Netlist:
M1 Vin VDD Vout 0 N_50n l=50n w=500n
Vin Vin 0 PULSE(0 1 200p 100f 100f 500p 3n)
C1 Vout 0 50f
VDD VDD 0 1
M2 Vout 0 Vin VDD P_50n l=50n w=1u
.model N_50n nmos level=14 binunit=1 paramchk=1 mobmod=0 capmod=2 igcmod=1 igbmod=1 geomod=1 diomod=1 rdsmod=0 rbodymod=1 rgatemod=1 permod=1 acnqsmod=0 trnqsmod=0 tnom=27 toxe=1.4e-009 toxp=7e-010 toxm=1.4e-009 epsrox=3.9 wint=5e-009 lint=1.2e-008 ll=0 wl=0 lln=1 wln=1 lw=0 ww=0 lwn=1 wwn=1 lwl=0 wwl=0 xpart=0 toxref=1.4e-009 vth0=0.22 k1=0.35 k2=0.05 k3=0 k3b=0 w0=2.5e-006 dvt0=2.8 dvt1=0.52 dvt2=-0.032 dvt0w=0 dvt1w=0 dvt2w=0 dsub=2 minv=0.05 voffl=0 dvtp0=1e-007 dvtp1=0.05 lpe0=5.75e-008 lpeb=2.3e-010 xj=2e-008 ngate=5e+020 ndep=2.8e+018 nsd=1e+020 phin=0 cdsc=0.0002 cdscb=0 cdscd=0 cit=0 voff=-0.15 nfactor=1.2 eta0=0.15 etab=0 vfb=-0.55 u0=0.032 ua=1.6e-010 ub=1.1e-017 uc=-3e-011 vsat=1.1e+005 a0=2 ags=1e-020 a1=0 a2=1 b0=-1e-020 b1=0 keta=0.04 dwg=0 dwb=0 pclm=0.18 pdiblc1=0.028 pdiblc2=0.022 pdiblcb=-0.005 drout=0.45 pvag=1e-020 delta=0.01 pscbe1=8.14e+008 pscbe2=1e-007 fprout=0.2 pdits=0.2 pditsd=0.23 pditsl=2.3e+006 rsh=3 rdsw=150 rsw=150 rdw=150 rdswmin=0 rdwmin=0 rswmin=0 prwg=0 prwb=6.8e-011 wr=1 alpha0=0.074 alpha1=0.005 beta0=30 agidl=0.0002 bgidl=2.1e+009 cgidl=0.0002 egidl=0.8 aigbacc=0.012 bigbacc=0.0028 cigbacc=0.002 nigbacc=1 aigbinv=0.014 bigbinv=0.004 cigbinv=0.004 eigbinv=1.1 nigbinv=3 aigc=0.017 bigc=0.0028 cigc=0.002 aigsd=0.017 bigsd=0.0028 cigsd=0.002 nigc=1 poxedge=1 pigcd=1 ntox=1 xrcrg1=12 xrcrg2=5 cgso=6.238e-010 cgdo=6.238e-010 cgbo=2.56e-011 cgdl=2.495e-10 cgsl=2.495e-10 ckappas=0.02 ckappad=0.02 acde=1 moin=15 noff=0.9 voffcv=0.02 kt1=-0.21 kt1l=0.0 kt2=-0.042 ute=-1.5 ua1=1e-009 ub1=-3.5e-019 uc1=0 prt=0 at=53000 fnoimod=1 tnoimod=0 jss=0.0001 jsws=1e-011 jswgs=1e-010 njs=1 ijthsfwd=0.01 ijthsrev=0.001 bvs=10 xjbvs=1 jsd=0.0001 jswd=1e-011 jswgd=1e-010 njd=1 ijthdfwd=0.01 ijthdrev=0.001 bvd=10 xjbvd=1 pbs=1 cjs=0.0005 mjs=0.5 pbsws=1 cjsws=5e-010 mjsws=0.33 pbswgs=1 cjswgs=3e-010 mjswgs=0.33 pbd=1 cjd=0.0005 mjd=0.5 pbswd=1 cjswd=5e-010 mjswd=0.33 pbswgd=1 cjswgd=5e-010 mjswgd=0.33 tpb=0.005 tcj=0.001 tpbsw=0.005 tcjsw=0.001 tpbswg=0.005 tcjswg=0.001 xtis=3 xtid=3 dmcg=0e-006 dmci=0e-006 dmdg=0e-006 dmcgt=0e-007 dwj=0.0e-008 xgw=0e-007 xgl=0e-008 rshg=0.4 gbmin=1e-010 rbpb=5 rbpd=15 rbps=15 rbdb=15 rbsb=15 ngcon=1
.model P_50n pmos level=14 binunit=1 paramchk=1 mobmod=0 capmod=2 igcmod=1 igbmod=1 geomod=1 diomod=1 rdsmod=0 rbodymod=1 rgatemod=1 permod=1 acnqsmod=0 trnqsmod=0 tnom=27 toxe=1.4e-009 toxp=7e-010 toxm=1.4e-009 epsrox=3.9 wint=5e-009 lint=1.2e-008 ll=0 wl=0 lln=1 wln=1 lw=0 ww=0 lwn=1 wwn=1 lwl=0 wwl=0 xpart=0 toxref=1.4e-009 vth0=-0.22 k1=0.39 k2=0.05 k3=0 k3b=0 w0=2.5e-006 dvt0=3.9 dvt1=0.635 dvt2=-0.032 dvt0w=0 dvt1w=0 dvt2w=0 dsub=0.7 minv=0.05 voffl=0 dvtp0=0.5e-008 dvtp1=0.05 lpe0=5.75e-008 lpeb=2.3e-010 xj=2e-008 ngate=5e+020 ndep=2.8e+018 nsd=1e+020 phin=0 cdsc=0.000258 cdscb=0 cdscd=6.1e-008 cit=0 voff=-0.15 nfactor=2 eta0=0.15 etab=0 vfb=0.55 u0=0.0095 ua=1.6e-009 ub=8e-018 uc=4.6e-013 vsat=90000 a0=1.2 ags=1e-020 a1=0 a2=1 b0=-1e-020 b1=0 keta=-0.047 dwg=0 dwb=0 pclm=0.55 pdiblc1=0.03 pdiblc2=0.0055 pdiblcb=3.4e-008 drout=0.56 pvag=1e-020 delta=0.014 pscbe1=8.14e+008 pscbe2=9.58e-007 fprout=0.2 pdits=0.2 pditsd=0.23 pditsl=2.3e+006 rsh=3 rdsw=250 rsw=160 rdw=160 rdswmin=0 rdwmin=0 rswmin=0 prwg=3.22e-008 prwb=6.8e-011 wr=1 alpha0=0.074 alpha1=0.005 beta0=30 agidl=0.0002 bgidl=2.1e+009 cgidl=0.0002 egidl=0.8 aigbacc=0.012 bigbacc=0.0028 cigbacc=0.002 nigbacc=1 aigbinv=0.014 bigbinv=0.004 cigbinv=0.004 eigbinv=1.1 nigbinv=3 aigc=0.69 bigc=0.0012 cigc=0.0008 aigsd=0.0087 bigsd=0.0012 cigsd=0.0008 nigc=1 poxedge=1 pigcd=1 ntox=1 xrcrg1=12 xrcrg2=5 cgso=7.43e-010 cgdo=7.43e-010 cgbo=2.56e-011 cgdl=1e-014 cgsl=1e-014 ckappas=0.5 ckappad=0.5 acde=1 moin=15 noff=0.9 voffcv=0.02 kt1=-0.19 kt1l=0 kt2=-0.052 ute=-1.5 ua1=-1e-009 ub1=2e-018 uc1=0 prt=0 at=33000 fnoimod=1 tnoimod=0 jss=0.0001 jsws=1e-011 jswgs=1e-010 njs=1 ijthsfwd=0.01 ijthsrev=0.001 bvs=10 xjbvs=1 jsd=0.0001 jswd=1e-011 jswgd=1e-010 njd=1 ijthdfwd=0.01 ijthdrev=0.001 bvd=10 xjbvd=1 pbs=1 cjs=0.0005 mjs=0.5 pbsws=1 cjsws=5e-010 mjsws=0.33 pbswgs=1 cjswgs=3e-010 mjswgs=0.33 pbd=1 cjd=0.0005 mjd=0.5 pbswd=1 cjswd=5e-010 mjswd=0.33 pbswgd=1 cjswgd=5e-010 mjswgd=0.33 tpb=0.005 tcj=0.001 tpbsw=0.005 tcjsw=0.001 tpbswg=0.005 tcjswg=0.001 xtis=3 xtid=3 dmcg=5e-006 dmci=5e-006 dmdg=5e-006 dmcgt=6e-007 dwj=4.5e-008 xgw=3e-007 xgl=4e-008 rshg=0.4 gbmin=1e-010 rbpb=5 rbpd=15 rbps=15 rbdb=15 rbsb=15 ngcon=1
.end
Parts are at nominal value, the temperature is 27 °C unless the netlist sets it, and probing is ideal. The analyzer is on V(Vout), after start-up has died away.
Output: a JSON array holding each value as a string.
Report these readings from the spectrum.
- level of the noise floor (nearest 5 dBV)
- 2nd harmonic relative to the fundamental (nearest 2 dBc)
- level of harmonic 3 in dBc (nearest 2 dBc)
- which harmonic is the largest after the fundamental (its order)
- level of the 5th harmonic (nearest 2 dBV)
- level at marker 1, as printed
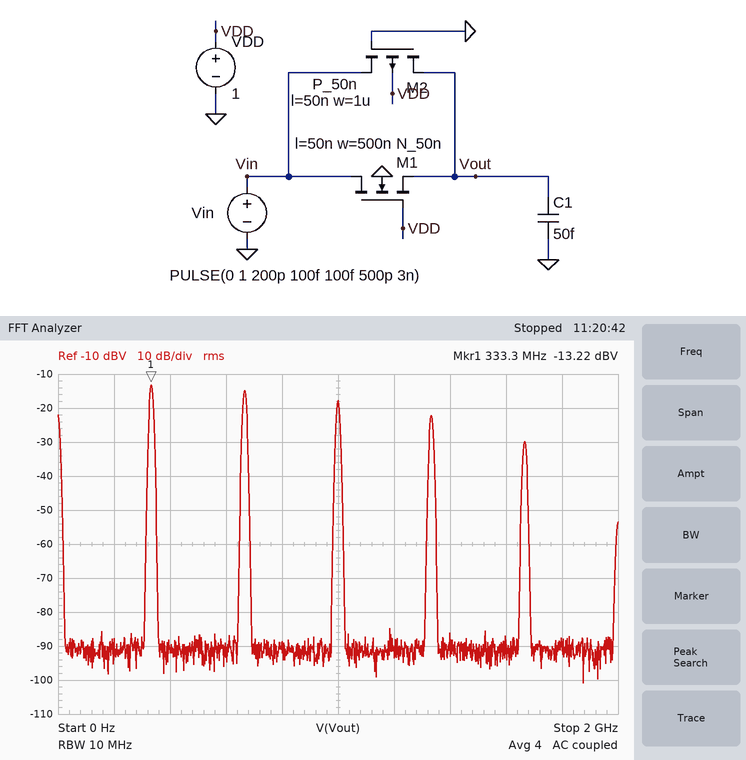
["-90 dBV", "-2 dBc", "-4 dBc", "2", "-30 dBV", "-13.22 dBV"]
